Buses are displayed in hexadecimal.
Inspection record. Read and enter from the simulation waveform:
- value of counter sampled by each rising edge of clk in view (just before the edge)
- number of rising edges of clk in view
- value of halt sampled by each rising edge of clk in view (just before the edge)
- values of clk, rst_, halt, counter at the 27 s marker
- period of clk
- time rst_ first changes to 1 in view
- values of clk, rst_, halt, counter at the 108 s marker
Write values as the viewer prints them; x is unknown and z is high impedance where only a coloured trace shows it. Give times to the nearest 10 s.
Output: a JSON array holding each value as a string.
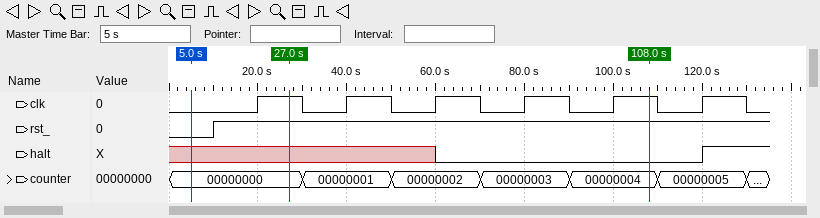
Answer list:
["00000000, 00000001, 00000002, 00000003, 00000004, 00000005", "6", "x x x 0 0 0", "clk=1, rst_=1, halt=x, counter=00000000", "20 s", "10 s", "clk=1, rst_=1, halt=0, counter=00000004"]
